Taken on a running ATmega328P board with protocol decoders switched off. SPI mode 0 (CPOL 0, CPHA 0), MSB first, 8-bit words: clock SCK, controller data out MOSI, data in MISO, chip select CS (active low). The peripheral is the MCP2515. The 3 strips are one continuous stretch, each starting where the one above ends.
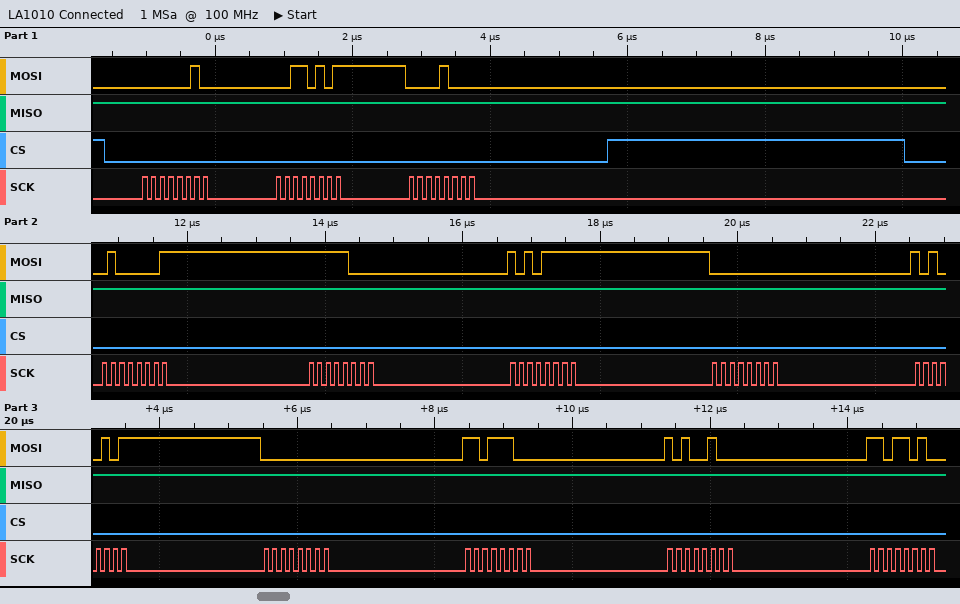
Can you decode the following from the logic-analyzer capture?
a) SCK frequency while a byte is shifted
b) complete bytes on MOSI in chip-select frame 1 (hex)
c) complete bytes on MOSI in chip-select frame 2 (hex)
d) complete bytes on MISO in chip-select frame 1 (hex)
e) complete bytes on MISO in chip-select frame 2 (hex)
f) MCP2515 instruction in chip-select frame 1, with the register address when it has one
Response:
8 MHz
02 35 08
41 F8 AF 00 A5 00 DC A4 DA
FF FF FF
FF FF FF FF FF FF FF FF FF
WRITE 0x35
